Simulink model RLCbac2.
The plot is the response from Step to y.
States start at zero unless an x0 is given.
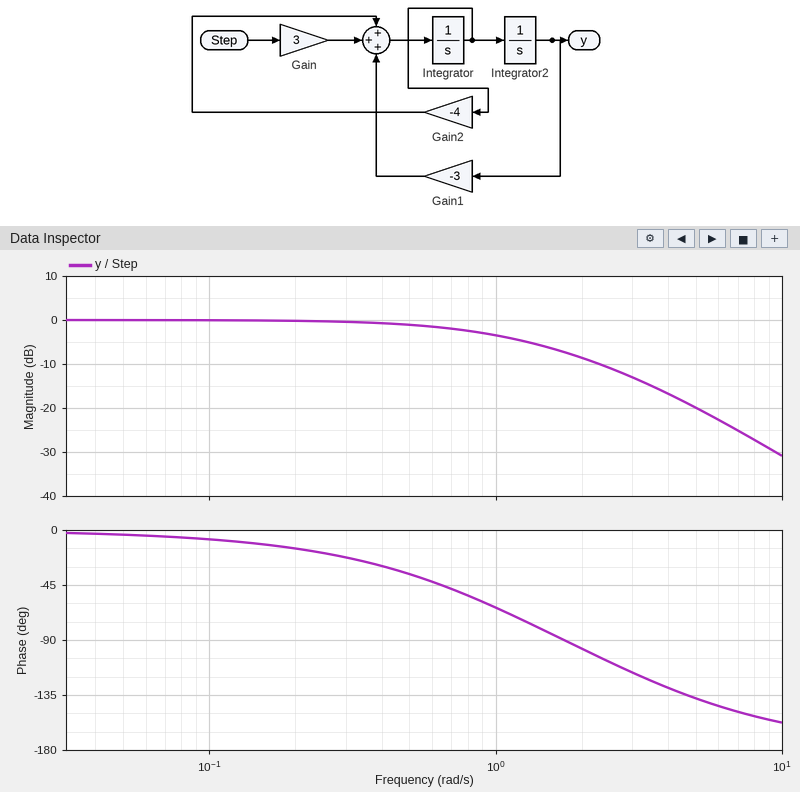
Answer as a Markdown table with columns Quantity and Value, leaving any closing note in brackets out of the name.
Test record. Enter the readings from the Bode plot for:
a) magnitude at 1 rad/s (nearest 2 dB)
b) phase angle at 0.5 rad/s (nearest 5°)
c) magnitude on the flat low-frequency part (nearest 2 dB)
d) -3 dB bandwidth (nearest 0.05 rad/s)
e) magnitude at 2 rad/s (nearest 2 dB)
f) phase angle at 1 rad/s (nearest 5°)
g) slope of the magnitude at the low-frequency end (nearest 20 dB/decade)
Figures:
| Quantity | Value |
|---|---|
| magnitude at 1 rad/s | -4 dB |
| phase angle at 0.5 rad/s | -35° |
| magnitude on the flat low-frequency part | 0 dB |
| -3 dB bandwidth | 0.90 rad/s |
| magnitude at 2 rad/s | -8 dB |
| phase angle at 1 rad/s | -65° |
| slope of the magnitude at the low-frequency end | 0 dB/decade |
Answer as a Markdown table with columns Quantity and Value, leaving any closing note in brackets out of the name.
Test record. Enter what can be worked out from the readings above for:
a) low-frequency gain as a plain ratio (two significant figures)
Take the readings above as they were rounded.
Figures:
| Quantity | Value |
|---|---|
| low-frequency gain as a plain ratio | 1.0 |
